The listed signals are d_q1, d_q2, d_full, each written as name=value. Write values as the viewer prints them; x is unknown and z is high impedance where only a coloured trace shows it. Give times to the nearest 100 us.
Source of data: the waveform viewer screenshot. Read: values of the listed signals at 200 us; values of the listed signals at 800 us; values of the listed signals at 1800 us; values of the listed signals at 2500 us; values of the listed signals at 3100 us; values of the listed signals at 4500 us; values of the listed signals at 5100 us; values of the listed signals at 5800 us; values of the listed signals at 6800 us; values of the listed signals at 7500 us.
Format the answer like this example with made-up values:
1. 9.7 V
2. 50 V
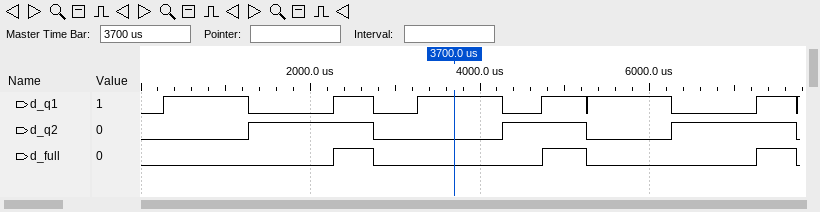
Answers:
1. d_q1=0, d_q2=0, d_full=0
2. d_q1=1, d_q2=0, d_full=0
3. d_q1=0, d_q2=1, d_full=0
4. d_q1=1, d_q2=1, d_full=1
5. d_q1=0, d_q2=0, d_full=0
6. d_q1=0, d_q2=1, d_full=0
7. d_q1=1, d_q2=1, d_full=1
8. d_q1=1, d_q2=0, d_full=0
9. d_q1=0, d_q2=1, d_full=0
10. d_q1=1, d_q2=1, d_full=1
